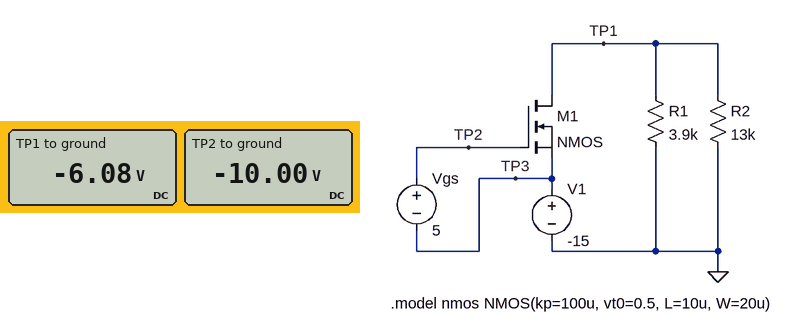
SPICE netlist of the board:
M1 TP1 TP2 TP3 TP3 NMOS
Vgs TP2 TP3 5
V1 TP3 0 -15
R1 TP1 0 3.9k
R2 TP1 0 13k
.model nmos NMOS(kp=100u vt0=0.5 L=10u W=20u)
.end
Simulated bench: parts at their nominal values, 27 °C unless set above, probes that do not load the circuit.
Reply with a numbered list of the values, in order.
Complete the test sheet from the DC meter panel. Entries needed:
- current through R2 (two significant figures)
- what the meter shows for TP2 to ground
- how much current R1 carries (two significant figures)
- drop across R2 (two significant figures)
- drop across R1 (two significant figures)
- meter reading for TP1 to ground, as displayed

1. 470 µA
2. -10.00 V
3. 1.6 mA
4. 6.1 V
5. 6.1 V
6. -6.08 V
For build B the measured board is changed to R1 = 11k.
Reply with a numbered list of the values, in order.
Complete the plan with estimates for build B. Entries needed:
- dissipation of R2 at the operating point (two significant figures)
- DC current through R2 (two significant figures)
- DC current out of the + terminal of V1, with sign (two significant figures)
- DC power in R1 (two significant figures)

1. 10 mW
2. 880 µA
3. -1.9 mA
4. 12 mW
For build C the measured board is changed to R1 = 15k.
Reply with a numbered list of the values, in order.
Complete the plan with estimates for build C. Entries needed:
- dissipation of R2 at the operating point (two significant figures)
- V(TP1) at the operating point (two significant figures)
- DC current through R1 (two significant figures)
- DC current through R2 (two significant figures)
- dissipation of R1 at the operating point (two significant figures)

1. 11 mW
2. -12 V
3. 810 µA
4. 940 µA
5. 9.9 mW
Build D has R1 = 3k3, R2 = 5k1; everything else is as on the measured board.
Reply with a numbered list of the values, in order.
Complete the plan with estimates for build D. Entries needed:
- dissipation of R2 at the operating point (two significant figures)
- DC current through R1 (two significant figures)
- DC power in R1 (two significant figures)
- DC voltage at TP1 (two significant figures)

1. 3.2 mW
2. 1.2 mA
3. 5.0 mW
4. -4.1 V
